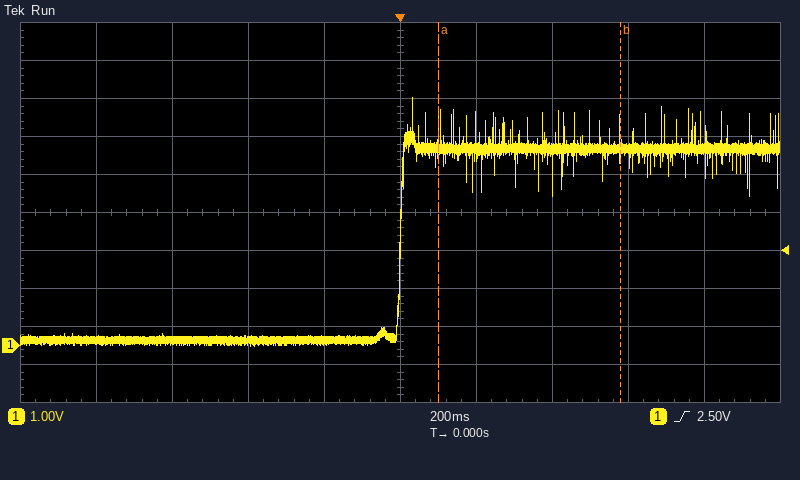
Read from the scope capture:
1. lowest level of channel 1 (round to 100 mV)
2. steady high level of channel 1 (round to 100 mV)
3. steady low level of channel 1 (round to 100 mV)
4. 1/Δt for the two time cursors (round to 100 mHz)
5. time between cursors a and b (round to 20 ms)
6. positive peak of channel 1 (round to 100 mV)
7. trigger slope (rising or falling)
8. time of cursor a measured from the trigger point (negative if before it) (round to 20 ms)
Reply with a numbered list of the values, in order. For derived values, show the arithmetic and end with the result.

1. 0.0 V
2. 5.2 V
3. 100 mV
4. 1 / 480 ms ≈ 2.1 Hz
5. 480 ms
6. 6.5 V
7. rising
8. +100 ms
